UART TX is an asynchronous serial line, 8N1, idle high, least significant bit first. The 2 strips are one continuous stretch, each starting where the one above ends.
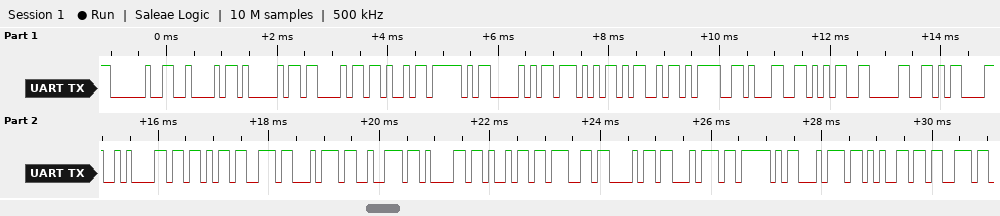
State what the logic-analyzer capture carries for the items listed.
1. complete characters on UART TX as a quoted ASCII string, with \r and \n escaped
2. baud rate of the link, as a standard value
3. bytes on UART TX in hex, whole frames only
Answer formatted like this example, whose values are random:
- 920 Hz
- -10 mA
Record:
- " BACK_PWM=150\r\n[straight_tes"
- 9600 baud
- 20 42 41 43 4B 5F 50 57 4D 3D 31 35 30 0D 0A 5B 73 74 72 61 69 67 68 74 5F 74 65 73
